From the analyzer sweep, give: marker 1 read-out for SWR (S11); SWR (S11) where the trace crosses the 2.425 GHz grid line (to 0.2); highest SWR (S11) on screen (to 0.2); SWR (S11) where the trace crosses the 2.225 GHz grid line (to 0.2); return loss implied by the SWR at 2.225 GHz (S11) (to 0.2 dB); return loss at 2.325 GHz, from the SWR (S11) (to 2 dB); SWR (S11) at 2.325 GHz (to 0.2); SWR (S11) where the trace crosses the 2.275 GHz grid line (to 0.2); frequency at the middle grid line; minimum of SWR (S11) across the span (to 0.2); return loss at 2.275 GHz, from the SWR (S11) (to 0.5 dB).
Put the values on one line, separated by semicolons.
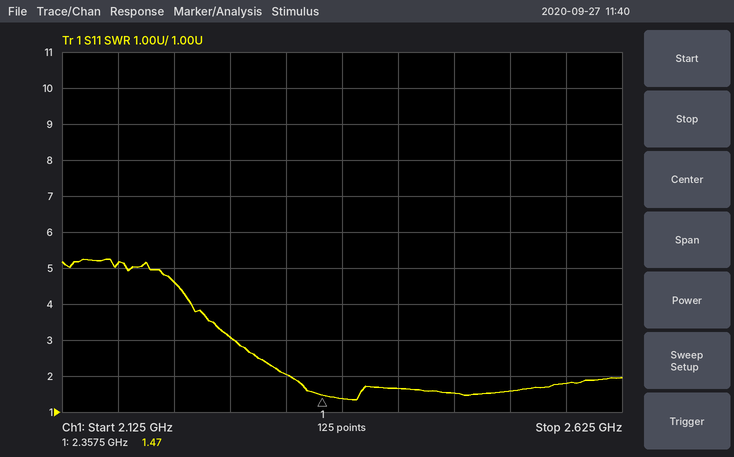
1.47; 1.6; 5.2; 4.6; 3.8 dB; 10 dB; 2.0; 3.0; 2.375 GHz; 1.4; 6.0 dB
